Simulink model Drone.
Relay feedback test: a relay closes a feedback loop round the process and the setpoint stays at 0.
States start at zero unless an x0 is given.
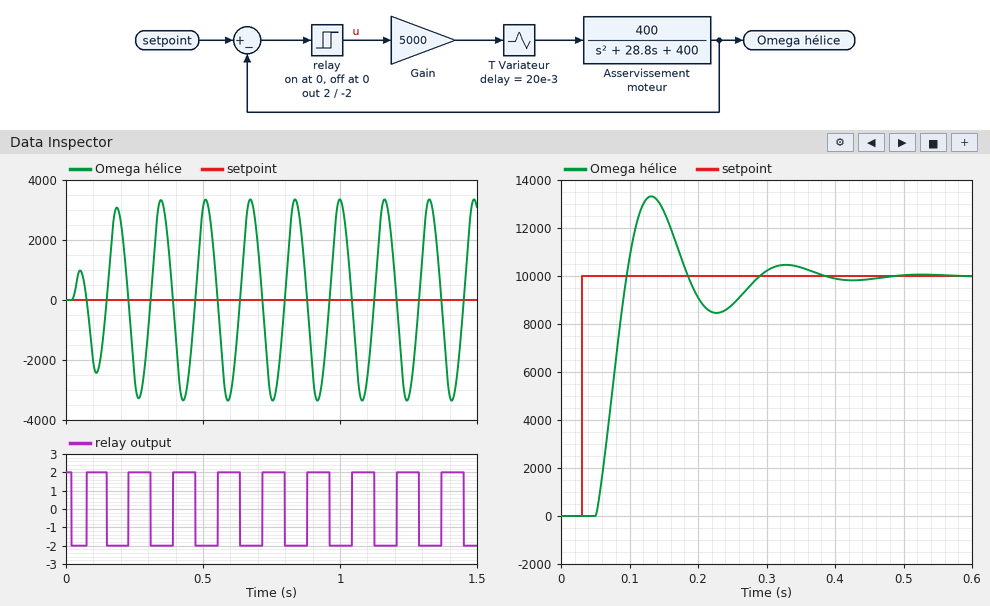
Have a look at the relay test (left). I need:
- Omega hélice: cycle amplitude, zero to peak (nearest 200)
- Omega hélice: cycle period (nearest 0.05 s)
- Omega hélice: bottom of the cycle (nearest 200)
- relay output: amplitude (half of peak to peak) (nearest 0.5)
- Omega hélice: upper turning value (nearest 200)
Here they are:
3400
0.15 s
-3400
2.0
3400
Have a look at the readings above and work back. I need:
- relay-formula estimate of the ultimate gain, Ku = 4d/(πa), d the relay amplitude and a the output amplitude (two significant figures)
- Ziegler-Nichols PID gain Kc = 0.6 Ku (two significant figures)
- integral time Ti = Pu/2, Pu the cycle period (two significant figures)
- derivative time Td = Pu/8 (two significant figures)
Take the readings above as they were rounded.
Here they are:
0.00075
0.00045
0.075 s
0.019 s
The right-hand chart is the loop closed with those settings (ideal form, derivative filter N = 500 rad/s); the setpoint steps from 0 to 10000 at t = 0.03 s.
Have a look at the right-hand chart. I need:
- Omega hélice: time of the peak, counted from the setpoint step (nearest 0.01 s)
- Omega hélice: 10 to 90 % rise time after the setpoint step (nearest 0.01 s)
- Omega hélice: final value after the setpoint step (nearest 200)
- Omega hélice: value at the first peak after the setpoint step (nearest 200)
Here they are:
0.10 s
0.03 s
10000
13400
